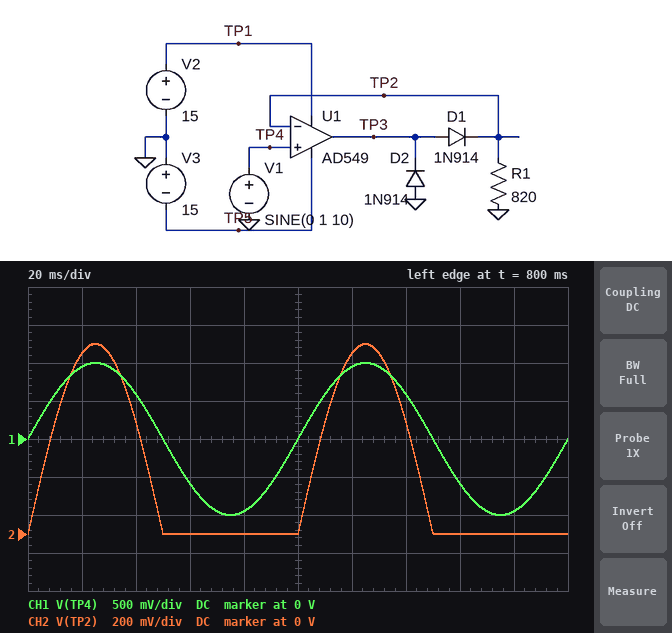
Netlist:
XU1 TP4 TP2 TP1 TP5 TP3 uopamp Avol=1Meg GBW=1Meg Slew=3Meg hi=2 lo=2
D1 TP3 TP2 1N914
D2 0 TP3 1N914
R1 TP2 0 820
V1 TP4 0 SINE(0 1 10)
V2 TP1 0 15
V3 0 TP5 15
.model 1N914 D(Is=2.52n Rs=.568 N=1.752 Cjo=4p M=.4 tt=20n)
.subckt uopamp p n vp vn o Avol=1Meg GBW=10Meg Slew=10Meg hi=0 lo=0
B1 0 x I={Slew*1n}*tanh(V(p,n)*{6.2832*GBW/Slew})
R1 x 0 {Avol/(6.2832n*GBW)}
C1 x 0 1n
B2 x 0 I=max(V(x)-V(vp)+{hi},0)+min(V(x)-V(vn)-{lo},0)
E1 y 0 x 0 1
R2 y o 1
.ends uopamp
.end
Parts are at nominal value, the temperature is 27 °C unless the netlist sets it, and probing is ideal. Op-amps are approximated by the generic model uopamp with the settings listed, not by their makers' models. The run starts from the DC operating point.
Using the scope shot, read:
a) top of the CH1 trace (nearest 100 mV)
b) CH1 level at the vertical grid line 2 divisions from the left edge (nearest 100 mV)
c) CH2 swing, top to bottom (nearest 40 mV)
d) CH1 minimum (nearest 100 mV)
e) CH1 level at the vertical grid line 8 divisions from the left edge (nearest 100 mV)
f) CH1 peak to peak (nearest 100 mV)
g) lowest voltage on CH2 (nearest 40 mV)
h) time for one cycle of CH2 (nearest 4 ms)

1.0 V
600 mV
1.00 V
-1.0 V
-600 mV
2.0 V
0 V
100 ms
